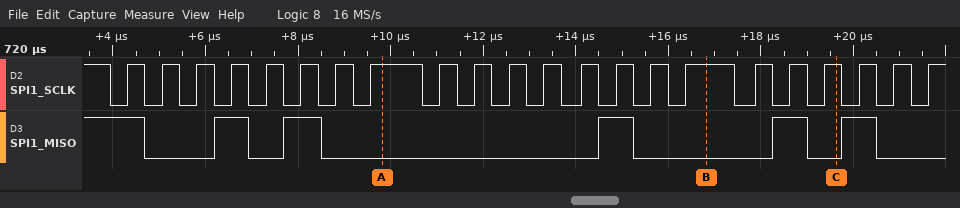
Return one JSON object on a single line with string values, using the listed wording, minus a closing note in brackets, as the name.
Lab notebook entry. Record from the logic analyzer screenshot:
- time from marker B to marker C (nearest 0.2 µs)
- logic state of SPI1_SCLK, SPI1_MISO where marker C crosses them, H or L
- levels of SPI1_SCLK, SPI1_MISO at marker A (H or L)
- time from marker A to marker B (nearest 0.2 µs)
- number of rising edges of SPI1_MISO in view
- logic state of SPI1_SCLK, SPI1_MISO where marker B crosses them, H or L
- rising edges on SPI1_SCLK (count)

{"time from marker B to marker C": "2.8 µs", "logic state of SPI1_SCLK, SPI1_MISO where marker C crosses them, H or L": "SPI1_SCLK=H, SPI1_MISO=L", "levels of SPI1_SCLK, SPI1_MISO at marker A": "SPI1_SCLK=H, SPI1_MISO=L", "time from marker A to marker B": "7 µs", "number of rising edges of SPI1_MISO in view": "5", "logic state of SPI1_SCLK, SPI1_MISO where marker B crosses them, H or L": "SPI1_SCLK=H, SPI1_MISO=L", "rising edges on SPI1_SCLK": "22"}
